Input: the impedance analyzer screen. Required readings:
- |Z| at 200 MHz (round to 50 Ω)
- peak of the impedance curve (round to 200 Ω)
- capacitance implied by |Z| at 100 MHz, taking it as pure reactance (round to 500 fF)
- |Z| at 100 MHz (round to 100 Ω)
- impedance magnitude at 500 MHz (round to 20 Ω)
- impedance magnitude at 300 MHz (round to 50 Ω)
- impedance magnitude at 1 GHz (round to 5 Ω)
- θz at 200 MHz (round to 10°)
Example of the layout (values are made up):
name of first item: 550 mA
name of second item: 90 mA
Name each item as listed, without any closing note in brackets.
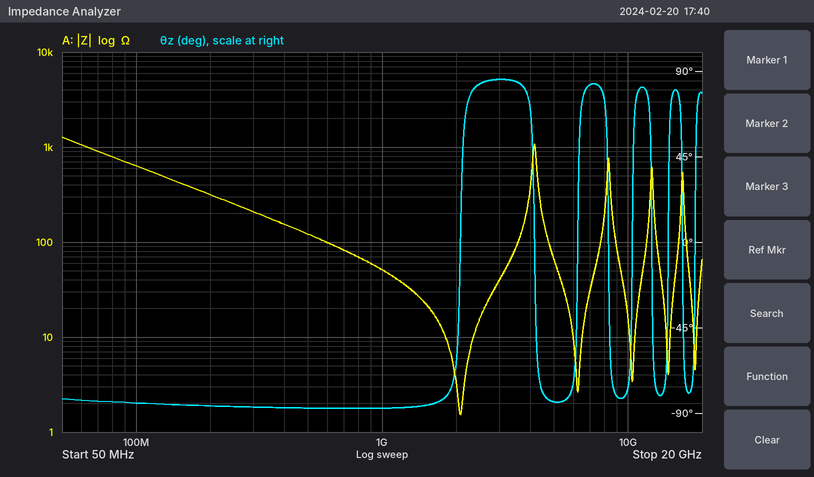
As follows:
|Z| at 200 MHz: 300 Ω
peak of the impedance curve: 1.2 kΩ
capacitance implied by |Z| at 100 MHz, taking it as pure reactance: 2.5 pF
|Z| at 100 MHz: 600 Ω
impedance magnitude at 500 MHz: 120 Ω
impedance magnitude at 300 MHz: 200 Ω
impedance magnitude at 1 GHz: 50 Ω
θz at 200 MHz: -90°
